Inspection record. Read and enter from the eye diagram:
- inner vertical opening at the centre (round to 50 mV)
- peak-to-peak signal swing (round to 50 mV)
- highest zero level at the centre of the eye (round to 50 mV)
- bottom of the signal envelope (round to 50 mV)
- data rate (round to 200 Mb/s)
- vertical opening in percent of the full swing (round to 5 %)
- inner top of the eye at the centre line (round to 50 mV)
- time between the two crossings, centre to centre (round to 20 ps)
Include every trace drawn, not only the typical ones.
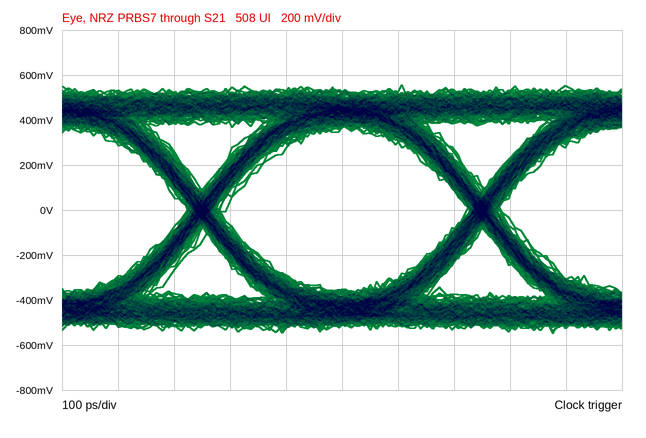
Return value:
700 mV
1.10 V
-350 mV
-550 mV
2.0 Gb/s
65 %
350 mV
500 ps
